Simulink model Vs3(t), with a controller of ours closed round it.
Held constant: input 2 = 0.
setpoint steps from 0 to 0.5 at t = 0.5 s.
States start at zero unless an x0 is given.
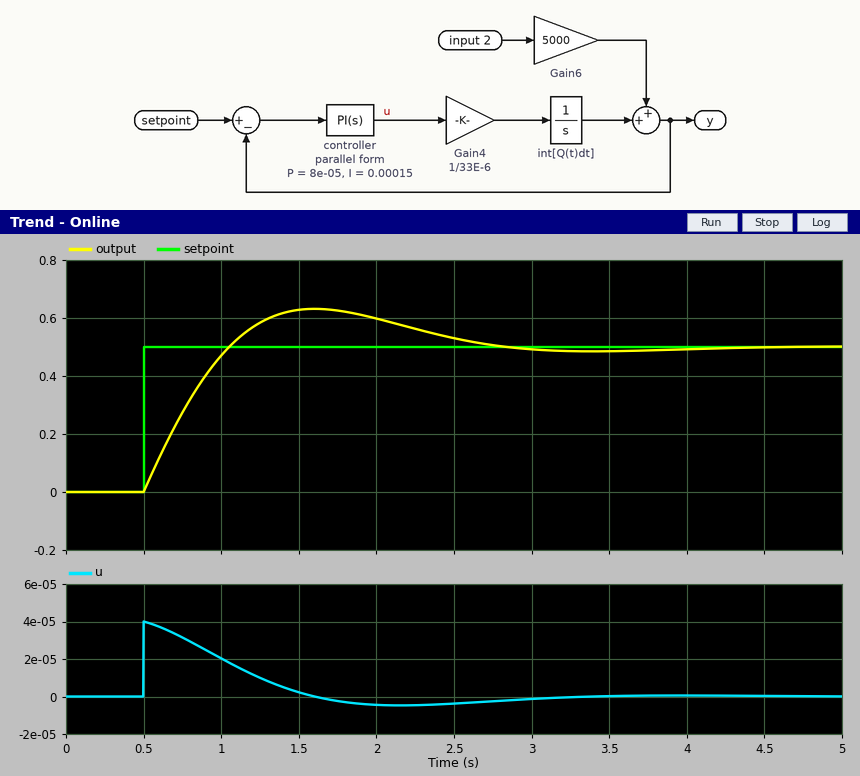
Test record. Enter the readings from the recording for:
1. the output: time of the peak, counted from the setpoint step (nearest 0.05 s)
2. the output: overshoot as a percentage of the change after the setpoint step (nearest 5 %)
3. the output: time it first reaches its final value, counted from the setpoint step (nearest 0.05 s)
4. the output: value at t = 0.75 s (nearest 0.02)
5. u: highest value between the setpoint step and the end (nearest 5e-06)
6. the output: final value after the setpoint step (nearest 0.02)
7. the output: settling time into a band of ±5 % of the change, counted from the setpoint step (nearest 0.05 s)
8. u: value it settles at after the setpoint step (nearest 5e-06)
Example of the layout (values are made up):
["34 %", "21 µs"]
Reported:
["1.10 s", "25 %", "0.55 s", "0.28", "0.000040", "0.50", "2.05 s", "0.000000"]
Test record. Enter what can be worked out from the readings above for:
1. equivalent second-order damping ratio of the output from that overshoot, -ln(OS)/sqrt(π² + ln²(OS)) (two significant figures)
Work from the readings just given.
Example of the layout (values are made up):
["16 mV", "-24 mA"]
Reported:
["0.40"]
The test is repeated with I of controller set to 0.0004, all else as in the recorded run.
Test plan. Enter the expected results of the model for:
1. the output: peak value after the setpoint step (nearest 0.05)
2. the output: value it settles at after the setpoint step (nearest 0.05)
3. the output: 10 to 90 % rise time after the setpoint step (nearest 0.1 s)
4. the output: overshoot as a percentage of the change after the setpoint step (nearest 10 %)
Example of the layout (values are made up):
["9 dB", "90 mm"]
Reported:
["0.70", "0.50", "0.3 s", "40 %"]
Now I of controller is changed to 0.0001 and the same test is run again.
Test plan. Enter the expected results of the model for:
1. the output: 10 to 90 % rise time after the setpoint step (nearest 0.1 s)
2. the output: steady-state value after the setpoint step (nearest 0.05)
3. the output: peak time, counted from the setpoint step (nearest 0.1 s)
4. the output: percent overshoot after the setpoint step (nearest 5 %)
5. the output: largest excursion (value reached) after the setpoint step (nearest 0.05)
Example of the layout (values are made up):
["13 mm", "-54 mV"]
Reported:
["0.5 s", "0.50", "1.3 s", "20 %", "0.60"]
